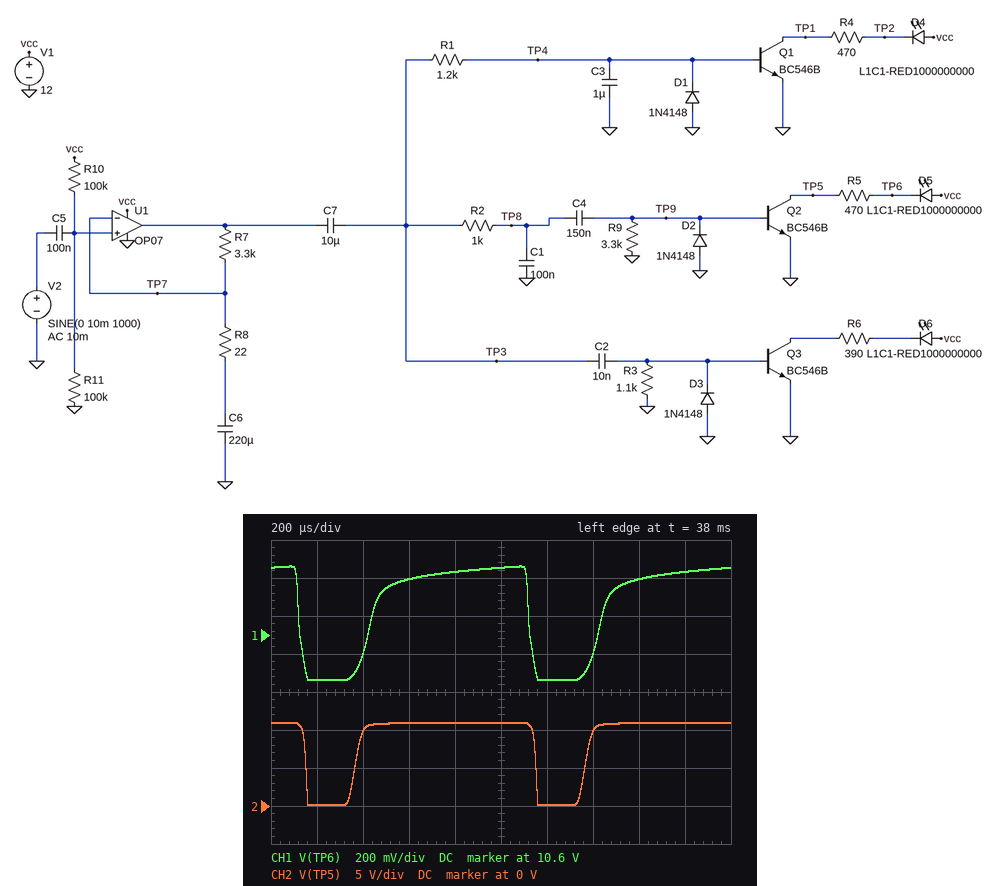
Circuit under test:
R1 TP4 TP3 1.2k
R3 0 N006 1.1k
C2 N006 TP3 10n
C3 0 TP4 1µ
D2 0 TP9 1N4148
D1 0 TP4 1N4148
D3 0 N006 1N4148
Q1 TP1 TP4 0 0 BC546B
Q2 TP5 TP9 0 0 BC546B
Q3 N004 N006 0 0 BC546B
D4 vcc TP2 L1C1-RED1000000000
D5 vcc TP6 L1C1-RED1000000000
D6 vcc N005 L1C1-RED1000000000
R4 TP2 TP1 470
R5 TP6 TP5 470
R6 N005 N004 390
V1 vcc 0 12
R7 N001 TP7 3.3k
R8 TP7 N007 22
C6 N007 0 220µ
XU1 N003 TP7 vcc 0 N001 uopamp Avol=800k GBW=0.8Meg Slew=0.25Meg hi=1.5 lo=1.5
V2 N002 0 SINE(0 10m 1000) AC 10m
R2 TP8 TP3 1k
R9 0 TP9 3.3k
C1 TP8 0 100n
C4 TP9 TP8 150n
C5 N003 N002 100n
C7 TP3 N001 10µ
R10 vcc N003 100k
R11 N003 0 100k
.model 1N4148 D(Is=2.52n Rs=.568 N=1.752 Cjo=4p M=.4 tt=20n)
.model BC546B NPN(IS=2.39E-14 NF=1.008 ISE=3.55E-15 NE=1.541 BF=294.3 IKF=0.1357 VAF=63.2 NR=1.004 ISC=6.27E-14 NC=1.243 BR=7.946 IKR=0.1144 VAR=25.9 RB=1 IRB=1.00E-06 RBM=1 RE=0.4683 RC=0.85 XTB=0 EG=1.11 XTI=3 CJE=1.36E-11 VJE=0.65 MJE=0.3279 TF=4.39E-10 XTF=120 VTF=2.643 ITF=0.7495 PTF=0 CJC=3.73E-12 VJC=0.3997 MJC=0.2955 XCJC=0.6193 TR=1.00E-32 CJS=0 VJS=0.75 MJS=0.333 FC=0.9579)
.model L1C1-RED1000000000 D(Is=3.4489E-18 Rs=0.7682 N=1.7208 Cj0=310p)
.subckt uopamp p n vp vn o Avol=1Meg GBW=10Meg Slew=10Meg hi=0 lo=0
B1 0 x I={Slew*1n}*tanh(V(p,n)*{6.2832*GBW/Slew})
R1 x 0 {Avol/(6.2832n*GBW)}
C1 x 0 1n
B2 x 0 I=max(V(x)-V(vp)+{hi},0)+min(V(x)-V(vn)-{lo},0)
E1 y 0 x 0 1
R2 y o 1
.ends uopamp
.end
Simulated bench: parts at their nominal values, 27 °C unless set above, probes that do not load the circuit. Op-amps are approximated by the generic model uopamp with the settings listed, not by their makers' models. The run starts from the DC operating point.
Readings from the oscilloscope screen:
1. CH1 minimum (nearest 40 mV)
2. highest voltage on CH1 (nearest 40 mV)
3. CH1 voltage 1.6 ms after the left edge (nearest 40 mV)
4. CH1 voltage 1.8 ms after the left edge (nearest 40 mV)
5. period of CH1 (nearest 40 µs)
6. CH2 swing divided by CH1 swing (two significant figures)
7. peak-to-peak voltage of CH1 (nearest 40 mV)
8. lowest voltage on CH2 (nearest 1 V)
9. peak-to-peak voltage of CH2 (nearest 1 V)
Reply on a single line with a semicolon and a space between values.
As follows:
10.36 V; 10.96 V; 10.88 V; 10.92 V; 1.00 ms; 18; 600 mV; 0 V; 11 V
